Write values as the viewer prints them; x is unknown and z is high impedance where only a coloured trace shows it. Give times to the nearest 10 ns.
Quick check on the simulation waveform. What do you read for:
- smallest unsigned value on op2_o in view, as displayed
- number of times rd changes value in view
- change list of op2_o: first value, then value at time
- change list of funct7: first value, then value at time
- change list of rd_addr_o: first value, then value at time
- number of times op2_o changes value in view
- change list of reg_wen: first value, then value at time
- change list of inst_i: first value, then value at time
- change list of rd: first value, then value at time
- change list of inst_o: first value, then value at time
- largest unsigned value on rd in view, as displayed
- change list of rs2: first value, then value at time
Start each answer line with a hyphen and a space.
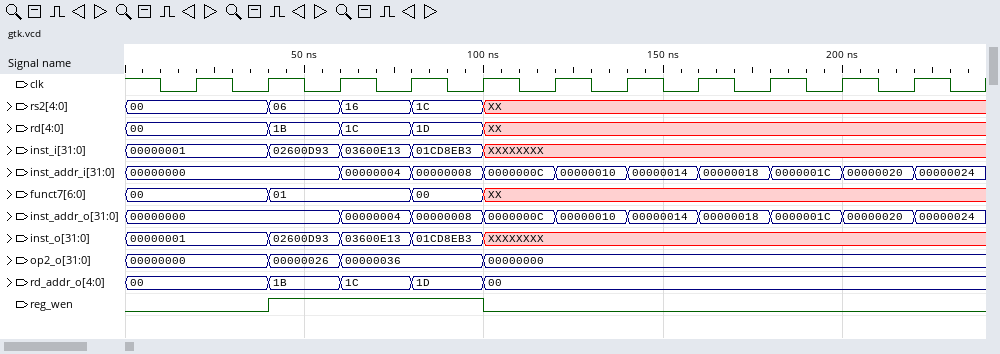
- 00000000
- 4
- 00000000, 00000026 at 40 ns, 00000036 at 60 ns, 00000000 at 100 ns
- 00, 01 at 40 ns, 00 at 80 ns, XX at 100 ns
- 00, 1B at 40 ns, 1C at 60 ns, 1D at 80 ns, 00 at 100 ns
- 3
- 0, 1 at 40 ns, 0 at 100 ns
- 00000001, 02600D93 at 40 ns, 03600E13 at 60 ns, 01CD8EB3 at 80 ns, XXXXXXXX at 100 ns
- 00, 1B at 40 ns, 1C at 60 ns, 1D at 80 ns, XX at 100 ns
- 00000001, 02600D93 at 40 ns, 03600E13 at 60 ns, 01CD8EB3 at 80 ns, XXXXXXXX at 100 ns
- 1D
- 00, 06 at 40 ns, 16 at 60 ns, 1C at 80 ns, XX at 100 ns
